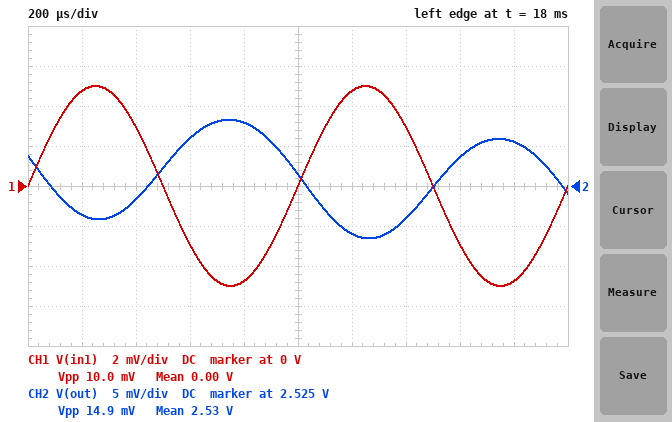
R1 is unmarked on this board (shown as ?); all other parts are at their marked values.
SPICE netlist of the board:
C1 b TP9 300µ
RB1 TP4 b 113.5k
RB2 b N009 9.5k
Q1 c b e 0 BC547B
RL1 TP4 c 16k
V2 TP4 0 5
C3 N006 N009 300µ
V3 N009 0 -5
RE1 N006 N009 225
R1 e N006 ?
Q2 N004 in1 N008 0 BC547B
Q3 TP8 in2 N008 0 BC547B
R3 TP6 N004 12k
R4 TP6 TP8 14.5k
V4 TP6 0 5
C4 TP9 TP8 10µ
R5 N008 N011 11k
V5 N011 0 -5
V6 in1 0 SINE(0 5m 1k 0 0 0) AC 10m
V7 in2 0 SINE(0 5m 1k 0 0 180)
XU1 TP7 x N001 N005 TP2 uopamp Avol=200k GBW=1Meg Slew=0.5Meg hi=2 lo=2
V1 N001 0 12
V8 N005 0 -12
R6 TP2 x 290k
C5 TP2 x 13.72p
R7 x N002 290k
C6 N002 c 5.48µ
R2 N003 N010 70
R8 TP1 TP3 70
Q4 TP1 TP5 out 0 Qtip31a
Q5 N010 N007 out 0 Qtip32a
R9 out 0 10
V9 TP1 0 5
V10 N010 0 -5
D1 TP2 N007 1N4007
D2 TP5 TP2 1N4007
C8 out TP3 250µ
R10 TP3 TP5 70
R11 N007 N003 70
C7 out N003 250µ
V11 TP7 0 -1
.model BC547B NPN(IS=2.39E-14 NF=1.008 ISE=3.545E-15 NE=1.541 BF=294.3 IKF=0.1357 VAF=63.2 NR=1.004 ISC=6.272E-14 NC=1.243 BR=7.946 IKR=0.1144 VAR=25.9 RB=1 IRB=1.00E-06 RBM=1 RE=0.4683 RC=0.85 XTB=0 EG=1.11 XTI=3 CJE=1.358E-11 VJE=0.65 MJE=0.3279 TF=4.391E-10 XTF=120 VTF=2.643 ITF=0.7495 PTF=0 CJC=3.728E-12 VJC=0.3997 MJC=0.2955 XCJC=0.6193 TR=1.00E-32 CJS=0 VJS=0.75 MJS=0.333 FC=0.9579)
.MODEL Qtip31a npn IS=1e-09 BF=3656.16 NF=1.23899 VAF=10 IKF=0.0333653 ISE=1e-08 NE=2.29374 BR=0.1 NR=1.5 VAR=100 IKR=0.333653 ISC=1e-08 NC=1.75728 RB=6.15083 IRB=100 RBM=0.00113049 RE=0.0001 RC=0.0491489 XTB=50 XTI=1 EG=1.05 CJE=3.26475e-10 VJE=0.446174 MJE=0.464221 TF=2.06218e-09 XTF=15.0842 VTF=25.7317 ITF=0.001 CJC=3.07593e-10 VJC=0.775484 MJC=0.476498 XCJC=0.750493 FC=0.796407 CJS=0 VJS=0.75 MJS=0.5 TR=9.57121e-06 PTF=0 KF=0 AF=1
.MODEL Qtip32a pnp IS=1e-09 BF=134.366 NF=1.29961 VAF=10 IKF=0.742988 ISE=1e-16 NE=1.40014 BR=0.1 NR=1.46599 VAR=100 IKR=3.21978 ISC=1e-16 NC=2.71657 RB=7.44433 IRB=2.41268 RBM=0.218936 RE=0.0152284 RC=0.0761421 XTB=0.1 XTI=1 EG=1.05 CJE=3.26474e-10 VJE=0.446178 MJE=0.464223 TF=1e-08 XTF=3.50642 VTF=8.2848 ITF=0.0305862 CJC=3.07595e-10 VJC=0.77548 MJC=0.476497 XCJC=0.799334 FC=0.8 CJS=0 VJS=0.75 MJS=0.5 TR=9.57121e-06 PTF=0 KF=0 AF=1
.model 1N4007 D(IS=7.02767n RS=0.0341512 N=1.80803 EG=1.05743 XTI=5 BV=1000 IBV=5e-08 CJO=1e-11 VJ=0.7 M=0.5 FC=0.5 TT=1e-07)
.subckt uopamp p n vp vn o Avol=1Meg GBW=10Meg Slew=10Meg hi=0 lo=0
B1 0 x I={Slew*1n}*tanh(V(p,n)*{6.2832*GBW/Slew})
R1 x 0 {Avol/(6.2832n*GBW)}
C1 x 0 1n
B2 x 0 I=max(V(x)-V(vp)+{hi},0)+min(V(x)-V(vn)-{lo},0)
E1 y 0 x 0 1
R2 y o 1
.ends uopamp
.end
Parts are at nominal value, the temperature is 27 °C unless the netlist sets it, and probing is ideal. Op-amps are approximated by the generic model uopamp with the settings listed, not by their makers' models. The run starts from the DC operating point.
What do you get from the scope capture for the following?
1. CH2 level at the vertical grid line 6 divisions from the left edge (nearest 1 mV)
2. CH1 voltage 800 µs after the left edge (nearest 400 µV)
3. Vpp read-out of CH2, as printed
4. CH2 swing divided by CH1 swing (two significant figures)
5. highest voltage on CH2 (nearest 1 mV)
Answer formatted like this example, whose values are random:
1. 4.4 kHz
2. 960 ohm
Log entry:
1. 2.519 V
2. -4.8 mV
3. 14.9 mV
4. 1.5
5. 2.533 V
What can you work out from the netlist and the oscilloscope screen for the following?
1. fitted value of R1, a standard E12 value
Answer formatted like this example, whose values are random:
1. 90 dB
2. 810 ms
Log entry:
1. 270 Ω
